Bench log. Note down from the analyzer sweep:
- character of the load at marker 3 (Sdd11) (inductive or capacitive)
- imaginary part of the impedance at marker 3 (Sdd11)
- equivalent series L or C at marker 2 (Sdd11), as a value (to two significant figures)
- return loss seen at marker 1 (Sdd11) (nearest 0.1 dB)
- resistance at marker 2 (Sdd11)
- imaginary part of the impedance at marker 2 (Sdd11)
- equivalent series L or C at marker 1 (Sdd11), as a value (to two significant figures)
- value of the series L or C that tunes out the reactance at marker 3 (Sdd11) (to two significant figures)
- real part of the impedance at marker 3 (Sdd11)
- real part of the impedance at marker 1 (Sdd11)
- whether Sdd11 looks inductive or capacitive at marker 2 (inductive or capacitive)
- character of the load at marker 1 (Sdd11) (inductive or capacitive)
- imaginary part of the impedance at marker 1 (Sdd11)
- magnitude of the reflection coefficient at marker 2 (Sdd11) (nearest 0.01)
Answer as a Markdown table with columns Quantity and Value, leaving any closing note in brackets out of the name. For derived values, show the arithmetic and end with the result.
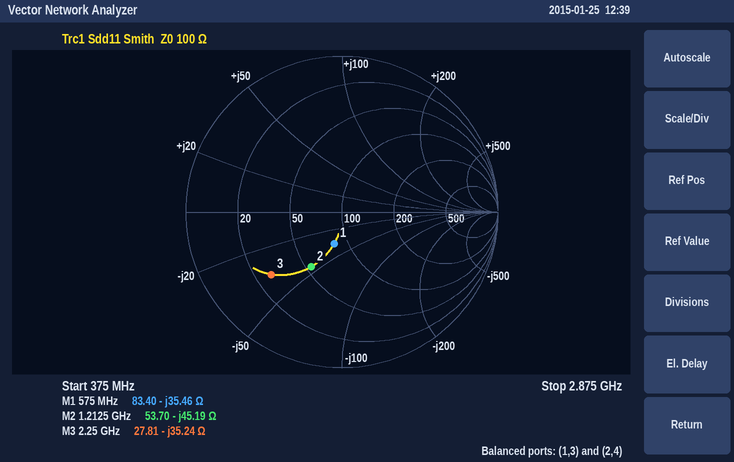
| Quantity | Value |
|---|---|
| character of the load at marker 3 (Sdd11) | capacitive |
| imaginary part of the impedance at marker 3 | -35.24 Ω |
| equivalent series L or C at marker 2 (Sdd11), as a value | C = 1/(2π × 1.2125 GHz × 45.19 Ω) ≈ 2.9 pF |
| return loss seen at marker 1 (Sdd11) | 13.6 dB |
| resistance at marker 2 | 53.70 Ω |
| imaginary part of the impedance at marker 2 | -45.19 Ω |
| equivalent series L or C at marker 1 (Sdd11), as a value | C = 1/(2π × 575 MHz × 35.46 Ω) ≈ 7.8 pF |
| value of the series L or C that tunes out the reactance at marker 3 (Sdd11) | L = 35.24 Ω/(2π × 2.25 GHz) ≈ 2.5 nH |
| real part of the impedance at marker 3 | 27.81 Ω |
| real part of the impedance at marker 1 | 83.40 Ω |
| whether Sdd11 looks inductive or capacitive at marker 2 | capacitive |
| character of the load at marker 1 (Sdd11) | capacitive |
| imaginary part of the impedance at marker 1 | -35.46 Ω |
| magnitude of the reflection coefficient at marker 2 (Sdd11) | 0.40 |
